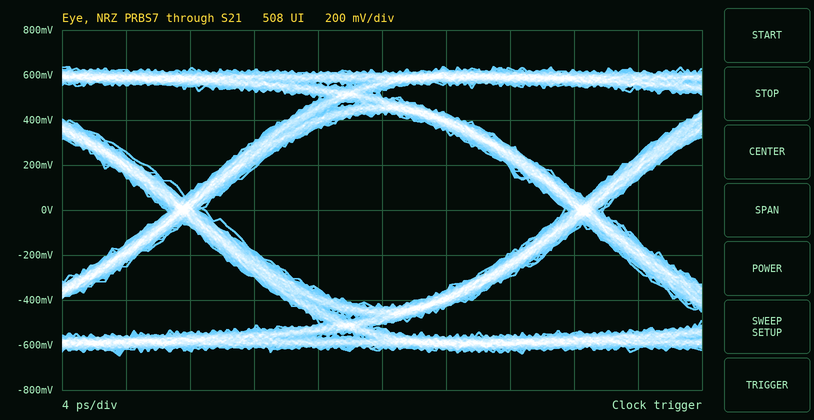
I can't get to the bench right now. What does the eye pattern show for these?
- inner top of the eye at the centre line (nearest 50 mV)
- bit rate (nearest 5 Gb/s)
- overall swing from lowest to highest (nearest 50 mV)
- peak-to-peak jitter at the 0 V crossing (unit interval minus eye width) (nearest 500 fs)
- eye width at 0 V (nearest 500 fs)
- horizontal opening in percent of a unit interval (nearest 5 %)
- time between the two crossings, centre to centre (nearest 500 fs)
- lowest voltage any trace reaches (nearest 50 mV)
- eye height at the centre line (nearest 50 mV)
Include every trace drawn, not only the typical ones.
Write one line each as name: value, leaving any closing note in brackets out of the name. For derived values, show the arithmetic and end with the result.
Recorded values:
inner top of the eye at the centre line: 450 mV
bit rate: 40 Gb/s
overall swing from lowest to highest: 1.30 V
peak-to-peak jitter at the 0 V crossing (unit interval minus eye width): 2.5 ps
eye width at 0 V: 22.5 ps
horizontal opening in percent of a unit interval: 22.5 ps / 25.0 ps ≈ 90 %
time between the two crossings, centre to centre: 25.0 ps
lowest voltage any trace reaches: -650 mV
eye height at the centre line: 850 mV
